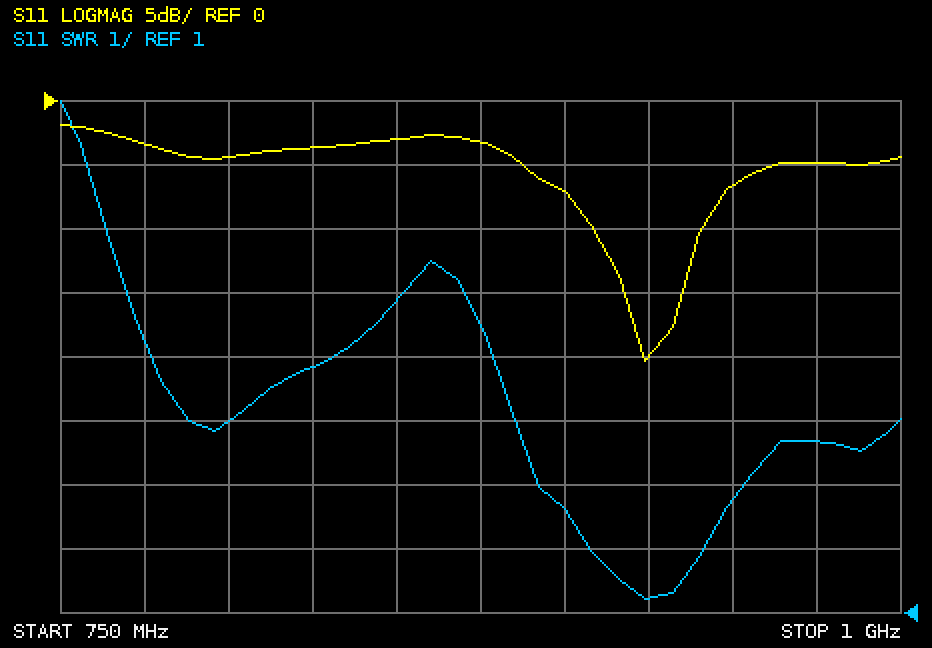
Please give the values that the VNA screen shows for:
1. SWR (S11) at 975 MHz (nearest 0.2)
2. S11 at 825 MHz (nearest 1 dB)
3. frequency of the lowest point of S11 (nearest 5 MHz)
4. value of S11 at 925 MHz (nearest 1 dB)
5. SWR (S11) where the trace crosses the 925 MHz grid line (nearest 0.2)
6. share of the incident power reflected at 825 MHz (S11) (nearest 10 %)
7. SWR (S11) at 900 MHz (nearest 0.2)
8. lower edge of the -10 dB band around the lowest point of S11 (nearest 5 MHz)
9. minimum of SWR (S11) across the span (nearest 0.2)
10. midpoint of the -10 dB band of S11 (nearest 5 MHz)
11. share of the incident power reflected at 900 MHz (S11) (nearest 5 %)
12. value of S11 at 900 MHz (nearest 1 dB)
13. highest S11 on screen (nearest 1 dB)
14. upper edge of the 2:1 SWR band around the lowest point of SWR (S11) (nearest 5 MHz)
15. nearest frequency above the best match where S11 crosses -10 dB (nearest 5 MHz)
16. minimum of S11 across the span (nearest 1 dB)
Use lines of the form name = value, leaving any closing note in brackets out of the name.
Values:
SWR (S11) at 975 MHz = 3.6
S11 at 825 MHz = -4 dB
frequency of the lowest point of S11 = 925 MHz
value of S11 at 925 MHz = -20 dB
SWR (S11) where the trace crosses the 925 MHz grid line = 1.2
share of the incident power reflected at 825 MHz (S11) = 40 %
SWR (S11) at 900 MHz = 2.6
lower edge of the -10 dB band around the lowest point of S11 = 910 MHz
minimum of SWR (S11) across the span = 1.2
midpoint of the -10 dB band of S11 = 925 MHz
share of the incident power reflected at 900 MHz (S11) = 20 %
value of S11 at 900 MHz = -7 dB
highest S11 on screen = -2 dB
upper edge of the 2:1 SWR band around the lowest point of SWR (S11) = 940 MHz
nearest frequency above the best match where S11 crosses -10 dB = 940 MHz
minimum of S11 across the span = -20 dB
